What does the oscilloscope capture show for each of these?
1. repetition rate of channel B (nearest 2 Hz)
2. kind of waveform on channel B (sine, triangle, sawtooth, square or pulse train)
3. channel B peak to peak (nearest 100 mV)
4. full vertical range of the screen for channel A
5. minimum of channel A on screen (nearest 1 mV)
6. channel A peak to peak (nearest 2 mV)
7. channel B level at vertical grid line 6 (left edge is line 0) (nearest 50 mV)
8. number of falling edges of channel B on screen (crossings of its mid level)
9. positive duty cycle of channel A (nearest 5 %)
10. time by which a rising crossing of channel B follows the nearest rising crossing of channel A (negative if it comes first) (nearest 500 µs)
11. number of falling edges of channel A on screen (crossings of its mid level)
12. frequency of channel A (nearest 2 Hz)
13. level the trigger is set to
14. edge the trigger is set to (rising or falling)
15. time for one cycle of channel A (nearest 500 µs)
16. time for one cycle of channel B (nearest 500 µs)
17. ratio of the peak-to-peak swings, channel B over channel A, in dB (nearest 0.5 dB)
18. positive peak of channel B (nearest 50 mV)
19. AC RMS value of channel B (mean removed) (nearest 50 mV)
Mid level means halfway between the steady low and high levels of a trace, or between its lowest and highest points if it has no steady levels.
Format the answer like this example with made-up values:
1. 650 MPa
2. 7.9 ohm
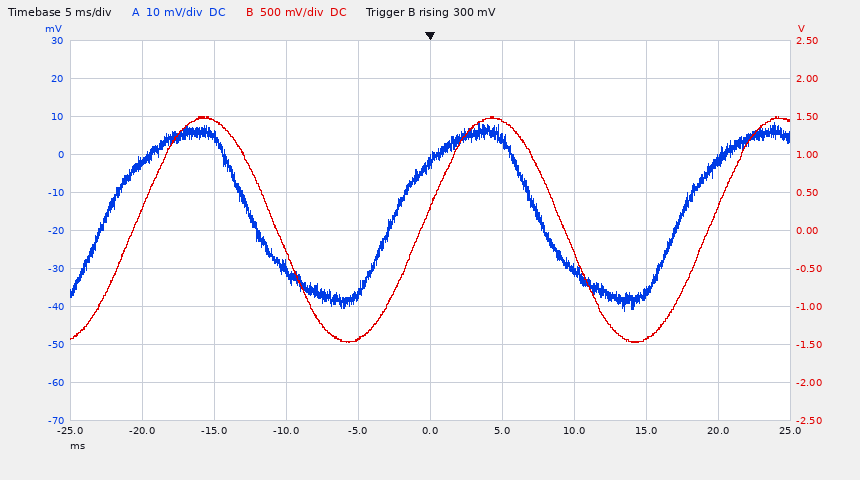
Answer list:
1. 50 Hz
2. sine
3. 3.00 V
4. 100 mV
5. -41 mV
6. 50 mV
7. 1.45 V
8. 2
9. 50 %
10. +2.0 ms
11. 2
12. 50 Hz
13. 300 mV
14. rising
15. 20.0 ms
16. 20.0 ms
17. 35.5 dB
18. 1.50 V
19. 1.05 V
